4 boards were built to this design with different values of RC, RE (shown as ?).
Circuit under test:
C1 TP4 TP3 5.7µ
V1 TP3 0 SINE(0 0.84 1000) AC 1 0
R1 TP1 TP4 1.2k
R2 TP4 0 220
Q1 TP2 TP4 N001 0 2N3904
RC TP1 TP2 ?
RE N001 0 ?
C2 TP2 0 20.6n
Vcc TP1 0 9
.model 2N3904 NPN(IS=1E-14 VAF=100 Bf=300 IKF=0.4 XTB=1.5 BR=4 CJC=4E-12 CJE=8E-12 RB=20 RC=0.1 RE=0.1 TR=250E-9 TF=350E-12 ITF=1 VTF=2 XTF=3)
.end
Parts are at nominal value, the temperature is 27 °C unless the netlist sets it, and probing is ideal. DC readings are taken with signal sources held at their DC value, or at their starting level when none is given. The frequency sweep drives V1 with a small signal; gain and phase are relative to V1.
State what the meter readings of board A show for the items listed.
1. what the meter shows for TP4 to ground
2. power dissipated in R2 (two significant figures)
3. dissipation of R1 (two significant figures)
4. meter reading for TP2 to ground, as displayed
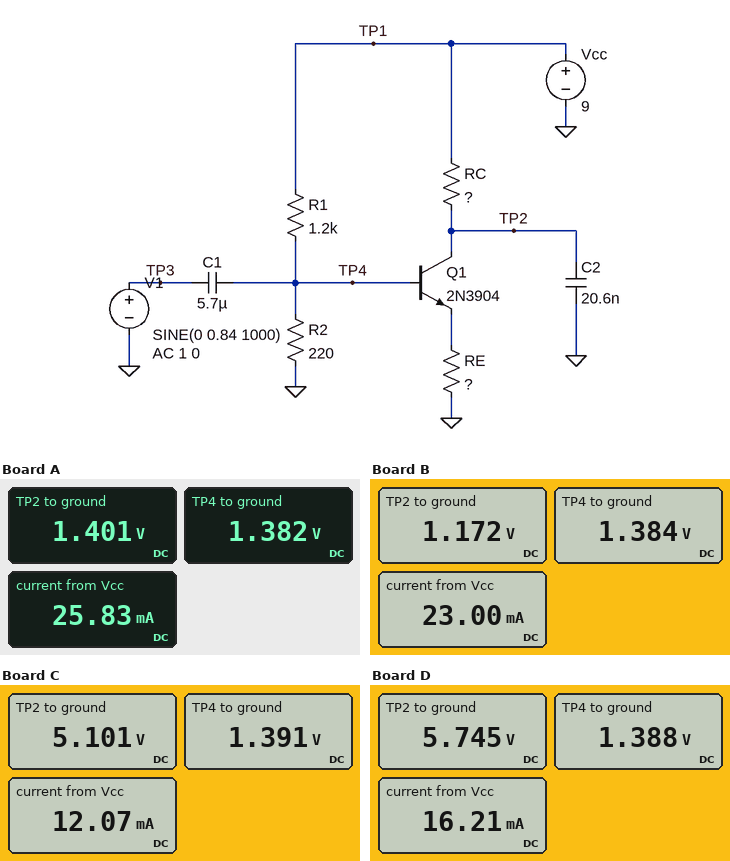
1.382 V
8.7 mW
48 mW
1.401 V
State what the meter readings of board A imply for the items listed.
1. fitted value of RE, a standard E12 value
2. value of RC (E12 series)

33 Ω
390 Ω
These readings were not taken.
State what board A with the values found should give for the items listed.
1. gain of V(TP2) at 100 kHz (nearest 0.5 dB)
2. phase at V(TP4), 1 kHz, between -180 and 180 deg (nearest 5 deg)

7.0 dB
10 deg
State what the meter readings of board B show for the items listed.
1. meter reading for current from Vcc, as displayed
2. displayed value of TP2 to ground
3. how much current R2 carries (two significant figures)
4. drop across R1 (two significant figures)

23.00 mA
1.172 V
6.3 mA
7.6 V
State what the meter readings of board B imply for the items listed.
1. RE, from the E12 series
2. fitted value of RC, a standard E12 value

39 Ω
470 Ω
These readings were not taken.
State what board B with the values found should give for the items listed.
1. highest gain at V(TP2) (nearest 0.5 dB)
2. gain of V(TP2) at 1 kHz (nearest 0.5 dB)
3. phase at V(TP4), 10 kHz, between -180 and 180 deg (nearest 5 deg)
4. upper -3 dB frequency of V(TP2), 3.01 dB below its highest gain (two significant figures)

21.0 dB
21.0 dB
0 deg
17 kHz
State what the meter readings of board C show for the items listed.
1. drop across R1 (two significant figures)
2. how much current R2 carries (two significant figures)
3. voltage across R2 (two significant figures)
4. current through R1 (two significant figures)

7.6 V
6.3 mA
1.4 V
6.3 mA
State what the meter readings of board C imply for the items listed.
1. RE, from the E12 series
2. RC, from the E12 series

120 Ω
680 Ω
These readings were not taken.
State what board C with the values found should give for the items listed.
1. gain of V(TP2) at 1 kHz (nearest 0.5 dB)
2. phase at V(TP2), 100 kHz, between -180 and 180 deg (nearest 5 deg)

14.5 dB
95 deg
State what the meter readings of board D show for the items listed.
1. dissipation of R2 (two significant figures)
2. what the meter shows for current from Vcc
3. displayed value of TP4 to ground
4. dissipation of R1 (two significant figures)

8.8 mW
16.21 mA
1.388 V
48 mW
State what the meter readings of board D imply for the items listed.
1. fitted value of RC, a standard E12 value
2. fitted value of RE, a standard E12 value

330 Ω
68 Ω
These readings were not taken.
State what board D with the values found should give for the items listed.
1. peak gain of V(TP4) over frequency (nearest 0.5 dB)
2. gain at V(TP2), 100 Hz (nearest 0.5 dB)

0 dB
8.0 dB
